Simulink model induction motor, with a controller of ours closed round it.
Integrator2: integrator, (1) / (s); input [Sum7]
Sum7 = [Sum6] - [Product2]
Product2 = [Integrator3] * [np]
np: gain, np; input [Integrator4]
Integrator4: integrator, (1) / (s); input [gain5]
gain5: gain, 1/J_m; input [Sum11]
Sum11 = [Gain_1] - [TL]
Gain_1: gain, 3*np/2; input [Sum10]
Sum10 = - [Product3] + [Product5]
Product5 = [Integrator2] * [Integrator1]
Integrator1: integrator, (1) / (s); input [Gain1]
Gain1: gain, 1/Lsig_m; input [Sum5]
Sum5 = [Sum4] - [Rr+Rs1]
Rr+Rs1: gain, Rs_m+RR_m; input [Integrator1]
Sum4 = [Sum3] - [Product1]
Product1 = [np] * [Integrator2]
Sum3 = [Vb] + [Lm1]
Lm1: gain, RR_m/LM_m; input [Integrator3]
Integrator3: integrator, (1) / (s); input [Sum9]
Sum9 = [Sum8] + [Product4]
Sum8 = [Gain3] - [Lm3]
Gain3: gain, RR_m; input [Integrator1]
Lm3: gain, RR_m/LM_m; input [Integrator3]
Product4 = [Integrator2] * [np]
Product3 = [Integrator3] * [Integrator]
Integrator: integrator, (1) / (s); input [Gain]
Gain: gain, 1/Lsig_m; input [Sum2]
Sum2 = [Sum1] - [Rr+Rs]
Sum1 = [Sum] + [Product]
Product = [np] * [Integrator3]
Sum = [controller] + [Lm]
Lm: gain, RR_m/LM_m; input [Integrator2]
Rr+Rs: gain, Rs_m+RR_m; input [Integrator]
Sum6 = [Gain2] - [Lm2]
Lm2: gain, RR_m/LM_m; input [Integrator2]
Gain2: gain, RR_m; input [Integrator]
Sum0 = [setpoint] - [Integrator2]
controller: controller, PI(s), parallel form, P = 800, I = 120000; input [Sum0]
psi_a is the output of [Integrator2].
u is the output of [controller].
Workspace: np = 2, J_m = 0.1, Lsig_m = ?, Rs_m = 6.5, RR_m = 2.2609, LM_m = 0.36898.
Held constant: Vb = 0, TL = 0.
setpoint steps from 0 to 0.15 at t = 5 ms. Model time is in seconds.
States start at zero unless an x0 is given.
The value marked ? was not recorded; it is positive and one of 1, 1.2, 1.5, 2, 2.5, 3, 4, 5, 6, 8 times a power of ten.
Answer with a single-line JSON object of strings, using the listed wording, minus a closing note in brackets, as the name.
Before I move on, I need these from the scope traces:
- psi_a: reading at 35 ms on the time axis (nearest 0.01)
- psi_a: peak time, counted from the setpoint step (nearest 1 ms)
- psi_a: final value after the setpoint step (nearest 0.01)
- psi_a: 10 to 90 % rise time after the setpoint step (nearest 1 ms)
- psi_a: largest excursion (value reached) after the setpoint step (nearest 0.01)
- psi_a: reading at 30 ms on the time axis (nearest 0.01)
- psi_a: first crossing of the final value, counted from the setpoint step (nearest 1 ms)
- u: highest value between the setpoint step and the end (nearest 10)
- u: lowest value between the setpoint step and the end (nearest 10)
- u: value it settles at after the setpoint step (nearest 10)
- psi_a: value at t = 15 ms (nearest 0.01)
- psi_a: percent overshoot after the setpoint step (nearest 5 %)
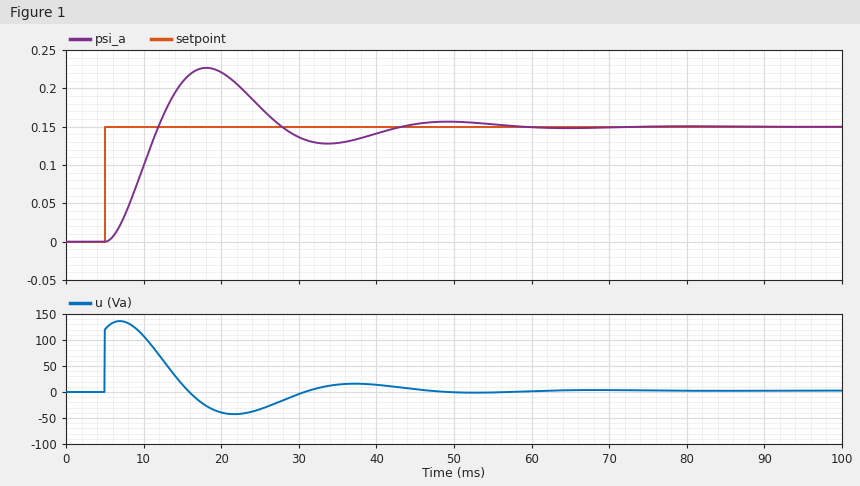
{"psi_a: reading at 35 ms on the time axis": "0.13", "psi_a: peak time, counted from the setpoint step": "13 ms", "psi_a: final value after the setpoint step": "0.15", "psi_a: 10 to 90 % rise time after the setpoint step": "5 ms", "psi_a: largest excursion (value reached) after the setpoint step": "0.23", "psi_a: reading at 30 ms on the time axis": "0.14", "psi_a: first crossing of the final value, counted from the setpoint step": "7 ms", "u: highest value between the setpoint step and the end": "140", "u: lowest value between the setpoint step and the end": "-40", "u: value it settles at after the setpoint step": "0", "psi_a: value at t = 15 ms": "0.21", "psi_a: percent overshoot after the setpoint step": "50 %"}
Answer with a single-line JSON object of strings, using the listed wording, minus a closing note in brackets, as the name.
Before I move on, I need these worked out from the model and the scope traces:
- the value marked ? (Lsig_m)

{"the value marked ?": "0.02"}
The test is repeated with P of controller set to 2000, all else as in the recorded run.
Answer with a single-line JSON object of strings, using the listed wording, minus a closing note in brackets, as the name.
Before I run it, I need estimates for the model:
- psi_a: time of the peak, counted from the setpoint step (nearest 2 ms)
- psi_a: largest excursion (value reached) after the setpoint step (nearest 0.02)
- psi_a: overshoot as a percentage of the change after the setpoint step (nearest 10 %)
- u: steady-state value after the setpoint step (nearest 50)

{"psi_a: time of the peak, counted from the setpoint step": "8 ms", "psi_a: largest excursion (value reached) after the setpoint step": "0.20", "psi_a: overshoot as a percentage of the change after the setpoint step": "30 %", "u: steady-state value after the setpoint step": "0"}
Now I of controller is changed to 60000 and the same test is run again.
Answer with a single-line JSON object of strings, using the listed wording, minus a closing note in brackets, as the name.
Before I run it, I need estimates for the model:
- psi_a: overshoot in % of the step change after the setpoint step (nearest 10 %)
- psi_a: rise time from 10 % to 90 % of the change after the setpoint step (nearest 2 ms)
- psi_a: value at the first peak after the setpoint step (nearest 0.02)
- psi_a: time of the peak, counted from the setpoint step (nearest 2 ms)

{"psi_a: overshoot in % of the step change after the setpoint step": "30 %", "psi_a: rise time from 10 % to 90 % of the change after the setpoint step": "6 ms", "psi_a: value at the first peak after the setpoint step": "0.20", "psi_a: time of the peak, counted from the setpoint step": "14 ms"}
